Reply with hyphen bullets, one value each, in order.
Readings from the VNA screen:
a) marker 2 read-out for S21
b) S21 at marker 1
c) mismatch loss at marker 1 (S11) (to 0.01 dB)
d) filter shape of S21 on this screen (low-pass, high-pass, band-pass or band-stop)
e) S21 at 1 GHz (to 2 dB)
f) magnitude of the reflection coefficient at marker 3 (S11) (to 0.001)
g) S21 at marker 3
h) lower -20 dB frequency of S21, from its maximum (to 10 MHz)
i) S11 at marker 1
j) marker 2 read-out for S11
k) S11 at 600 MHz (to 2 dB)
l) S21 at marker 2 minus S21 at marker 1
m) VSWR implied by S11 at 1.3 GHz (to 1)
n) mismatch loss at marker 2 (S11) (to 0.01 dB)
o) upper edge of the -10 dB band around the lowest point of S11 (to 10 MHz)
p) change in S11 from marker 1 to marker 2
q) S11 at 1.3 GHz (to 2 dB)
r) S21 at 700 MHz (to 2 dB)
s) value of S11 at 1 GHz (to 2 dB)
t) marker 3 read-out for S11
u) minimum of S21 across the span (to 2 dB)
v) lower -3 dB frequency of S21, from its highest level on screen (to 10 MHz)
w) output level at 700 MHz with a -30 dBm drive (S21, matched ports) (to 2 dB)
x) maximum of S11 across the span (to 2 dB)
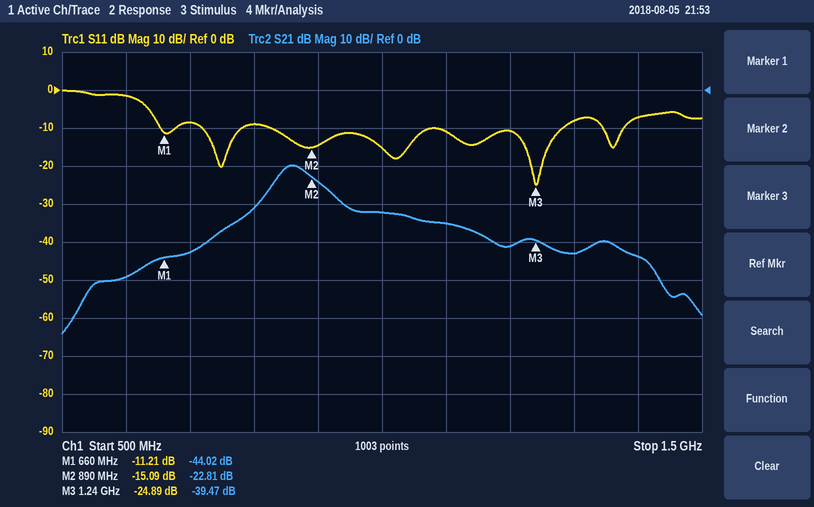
- -22.81 dB
- -44.02 dB
- 0.34 dB
- band-pass
- -32 dB
- 0.057
- -39.47 dB
- 730 MHz
- -11.21 dB
- -15.09 dB
- -2 dB
- 21.21 dB
- 2
- 0.14 dB
- 1.28 GHz
- -3.88 dB
- -8 dB
- -42 dB
- -16 dB
- -24.89 dB
- -64 dB
- 840 MHz
- -72 dBm
- 0 dB
